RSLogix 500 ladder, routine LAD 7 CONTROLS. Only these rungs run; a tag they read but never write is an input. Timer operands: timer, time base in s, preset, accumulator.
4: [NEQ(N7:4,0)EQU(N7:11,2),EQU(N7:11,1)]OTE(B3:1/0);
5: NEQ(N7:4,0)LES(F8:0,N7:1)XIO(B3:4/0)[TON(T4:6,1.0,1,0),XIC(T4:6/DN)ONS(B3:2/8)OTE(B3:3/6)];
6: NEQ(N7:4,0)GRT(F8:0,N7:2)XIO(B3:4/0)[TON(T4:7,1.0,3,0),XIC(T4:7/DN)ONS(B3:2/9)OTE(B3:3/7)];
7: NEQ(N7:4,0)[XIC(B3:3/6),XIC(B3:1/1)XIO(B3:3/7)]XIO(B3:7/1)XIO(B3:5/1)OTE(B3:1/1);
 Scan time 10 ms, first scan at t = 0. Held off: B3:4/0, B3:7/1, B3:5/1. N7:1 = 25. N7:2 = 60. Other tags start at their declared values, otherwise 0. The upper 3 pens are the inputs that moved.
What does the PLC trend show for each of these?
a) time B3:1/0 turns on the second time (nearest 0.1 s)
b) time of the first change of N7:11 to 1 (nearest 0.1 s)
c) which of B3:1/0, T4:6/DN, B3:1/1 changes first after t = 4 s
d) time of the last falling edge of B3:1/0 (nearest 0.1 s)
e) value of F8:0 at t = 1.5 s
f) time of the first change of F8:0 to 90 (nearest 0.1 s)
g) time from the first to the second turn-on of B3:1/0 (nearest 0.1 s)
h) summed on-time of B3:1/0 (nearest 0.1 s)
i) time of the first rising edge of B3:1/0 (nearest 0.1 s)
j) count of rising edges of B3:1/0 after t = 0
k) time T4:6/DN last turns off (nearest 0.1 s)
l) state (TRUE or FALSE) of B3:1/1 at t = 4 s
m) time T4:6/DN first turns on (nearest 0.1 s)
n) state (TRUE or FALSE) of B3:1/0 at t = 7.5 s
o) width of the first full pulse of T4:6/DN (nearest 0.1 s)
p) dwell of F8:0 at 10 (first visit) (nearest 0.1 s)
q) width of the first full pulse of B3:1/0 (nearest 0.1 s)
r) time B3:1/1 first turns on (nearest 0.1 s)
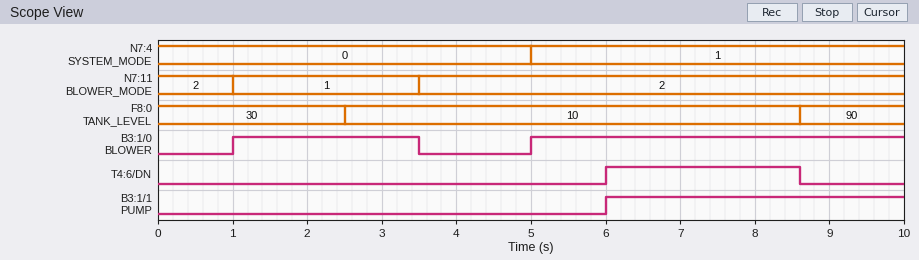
5.0 s
1.0 s
B3:1/0
3.5 s
30
8.6 s
4.0 s
7.5 s
1.0 s
2
8.6 s
FALSE
6.0 s
TRUE
2.6 s
6.1 s
2.5 s
6.0 s
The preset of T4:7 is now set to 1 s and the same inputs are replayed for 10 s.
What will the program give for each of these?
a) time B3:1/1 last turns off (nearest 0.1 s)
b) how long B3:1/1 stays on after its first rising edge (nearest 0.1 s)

9.6 s
3.6 s
